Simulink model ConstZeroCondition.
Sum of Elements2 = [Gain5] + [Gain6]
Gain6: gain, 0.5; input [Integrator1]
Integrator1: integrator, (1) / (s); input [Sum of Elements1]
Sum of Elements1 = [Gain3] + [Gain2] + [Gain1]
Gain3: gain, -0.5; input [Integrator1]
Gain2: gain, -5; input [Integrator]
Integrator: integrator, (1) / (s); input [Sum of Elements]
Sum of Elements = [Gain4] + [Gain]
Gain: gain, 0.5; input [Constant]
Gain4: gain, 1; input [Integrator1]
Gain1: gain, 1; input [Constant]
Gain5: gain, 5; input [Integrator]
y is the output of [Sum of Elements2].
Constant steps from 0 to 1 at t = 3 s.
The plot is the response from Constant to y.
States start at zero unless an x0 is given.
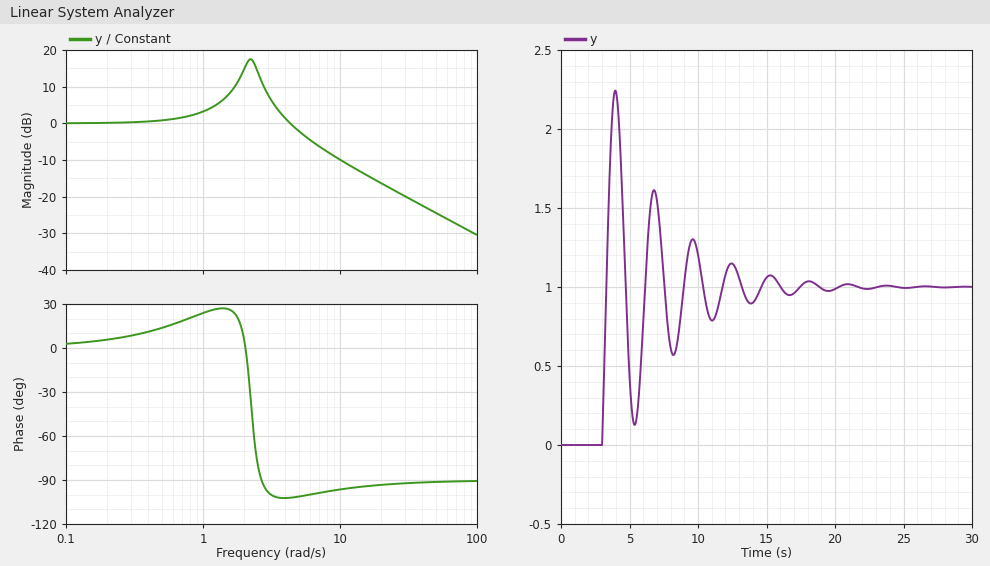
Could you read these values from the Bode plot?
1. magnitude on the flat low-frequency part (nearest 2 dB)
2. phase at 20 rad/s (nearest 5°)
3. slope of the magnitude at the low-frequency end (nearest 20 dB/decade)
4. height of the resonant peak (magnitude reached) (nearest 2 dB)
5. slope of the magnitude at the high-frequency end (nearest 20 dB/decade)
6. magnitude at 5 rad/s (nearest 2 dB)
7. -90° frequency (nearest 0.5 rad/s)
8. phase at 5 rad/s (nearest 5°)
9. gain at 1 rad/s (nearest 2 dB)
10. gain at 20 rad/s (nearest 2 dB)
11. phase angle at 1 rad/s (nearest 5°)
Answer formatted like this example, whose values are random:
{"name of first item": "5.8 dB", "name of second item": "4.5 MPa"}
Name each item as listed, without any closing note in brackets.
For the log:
{"magnitude on the flat low-frequency part": "0 dB", "phase at 20 rad/s": "-95°", "slope of the magnitude at the low-frequency end": "0 dB/decade", "height of the resonant peak (magnitude reached)": "18 dB", "slope of the magnitude at the high-frequency end": "-20 dB/decade", "magnitude at 5 rad/s": "-2 dB", "-90° frequency": "2.5 rad/s", "phase at 5 rad/s": "-100°", "gain at 1 rad/s": "4 dB", "gain at 20 rad/s": "-16 dB", "phase angle at 1 rad/s": "25°"}
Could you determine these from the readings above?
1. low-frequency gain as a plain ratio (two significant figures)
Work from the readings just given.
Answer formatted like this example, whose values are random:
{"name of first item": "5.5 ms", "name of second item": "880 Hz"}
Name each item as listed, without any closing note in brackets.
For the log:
{"low-frequency gain as a plain ratio": "1.0"}
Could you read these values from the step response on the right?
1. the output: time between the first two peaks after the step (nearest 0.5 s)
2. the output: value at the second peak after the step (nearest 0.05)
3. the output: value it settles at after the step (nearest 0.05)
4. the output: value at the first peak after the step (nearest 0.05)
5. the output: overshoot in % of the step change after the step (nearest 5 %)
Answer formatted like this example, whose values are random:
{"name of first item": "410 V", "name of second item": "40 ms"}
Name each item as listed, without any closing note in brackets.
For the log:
{"the output: time between the first two peaks after the step": "3.0 s", "the output: value at the second peak after the step": "1.60", "the output: value it settles at after the step": "1.00", "the output: value at the first peak after the step": "2.25", "the output: overshoot in % of the step change after the step": "125 %"}
